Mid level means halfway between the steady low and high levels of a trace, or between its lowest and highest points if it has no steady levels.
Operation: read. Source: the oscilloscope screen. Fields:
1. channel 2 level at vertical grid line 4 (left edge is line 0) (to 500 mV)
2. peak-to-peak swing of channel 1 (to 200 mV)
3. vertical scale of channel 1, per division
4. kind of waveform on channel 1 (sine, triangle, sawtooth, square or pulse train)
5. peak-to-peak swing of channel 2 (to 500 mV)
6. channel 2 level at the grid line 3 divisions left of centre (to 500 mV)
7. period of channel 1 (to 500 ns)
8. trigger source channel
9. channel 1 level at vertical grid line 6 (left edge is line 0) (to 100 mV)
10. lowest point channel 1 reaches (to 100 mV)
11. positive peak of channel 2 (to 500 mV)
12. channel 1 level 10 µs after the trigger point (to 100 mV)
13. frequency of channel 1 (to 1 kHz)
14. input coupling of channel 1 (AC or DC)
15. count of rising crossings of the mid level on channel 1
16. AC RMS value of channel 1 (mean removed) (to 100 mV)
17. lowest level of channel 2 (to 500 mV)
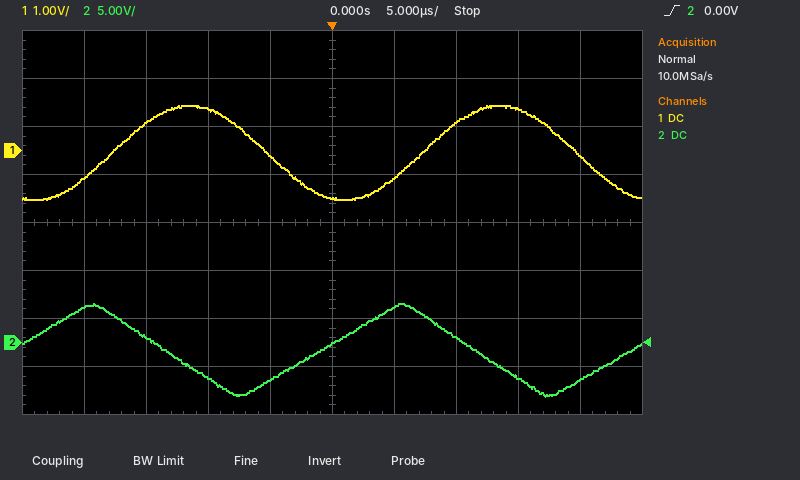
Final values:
-4.0 V
2.0 V
1 V
sine
9.5 V
500 mV
25.0 µs
channel 2
-600 mV
-1.0 V
4.0 V
600 mV
40 kHz
DC
2
700 mV
-5.5 V
